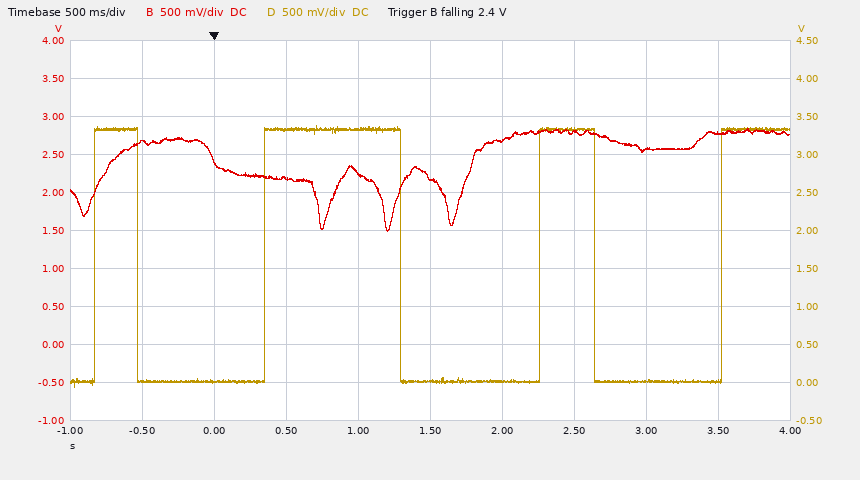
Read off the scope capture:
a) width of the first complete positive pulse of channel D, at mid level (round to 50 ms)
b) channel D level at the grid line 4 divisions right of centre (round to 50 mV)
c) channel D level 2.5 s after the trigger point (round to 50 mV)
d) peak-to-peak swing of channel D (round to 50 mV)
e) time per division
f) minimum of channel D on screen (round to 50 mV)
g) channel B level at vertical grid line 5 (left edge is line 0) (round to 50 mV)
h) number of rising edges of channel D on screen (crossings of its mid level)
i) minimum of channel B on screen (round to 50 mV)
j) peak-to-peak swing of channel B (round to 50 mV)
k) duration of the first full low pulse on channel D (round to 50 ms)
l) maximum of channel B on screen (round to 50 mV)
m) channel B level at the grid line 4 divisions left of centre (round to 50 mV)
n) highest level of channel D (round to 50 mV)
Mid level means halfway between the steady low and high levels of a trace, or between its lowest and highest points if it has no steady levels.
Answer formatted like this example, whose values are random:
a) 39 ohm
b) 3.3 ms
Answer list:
a) 300 ms
b) 0 mV
c) 3.35 V
d) 3.45 V
e) 500 ms
f) -50 mV
g) 2.20 V
h) 4
i) 1.50 V
j) 1.35 V
k) 900 ms
l) 2.85 V
m) 2.65 V
n) 3.40 V
